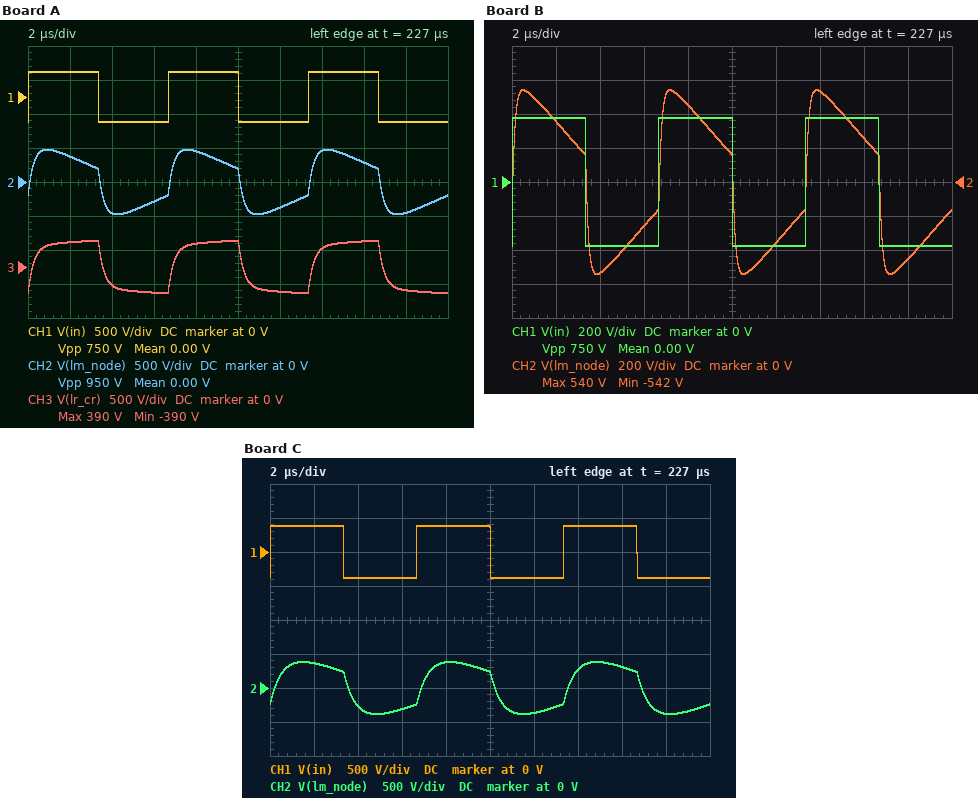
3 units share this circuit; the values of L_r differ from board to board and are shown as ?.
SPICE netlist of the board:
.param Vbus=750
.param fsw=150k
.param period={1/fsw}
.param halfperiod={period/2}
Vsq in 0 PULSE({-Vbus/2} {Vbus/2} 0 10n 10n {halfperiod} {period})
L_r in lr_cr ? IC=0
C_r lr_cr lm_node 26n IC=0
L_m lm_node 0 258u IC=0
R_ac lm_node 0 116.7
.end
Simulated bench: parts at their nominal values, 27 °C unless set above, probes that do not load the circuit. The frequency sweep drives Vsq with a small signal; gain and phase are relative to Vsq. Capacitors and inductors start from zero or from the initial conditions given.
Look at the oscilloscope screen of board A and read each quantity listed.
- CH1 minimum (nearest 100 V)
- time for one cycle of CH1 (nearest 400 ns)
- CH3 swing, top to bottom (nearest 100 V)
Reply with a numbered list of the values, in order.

1. -400 V
2. 6.8 µs
3. 800 V
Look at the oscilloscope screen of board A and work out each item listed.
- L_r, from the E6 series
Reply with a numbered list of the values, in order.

1. 33 µH
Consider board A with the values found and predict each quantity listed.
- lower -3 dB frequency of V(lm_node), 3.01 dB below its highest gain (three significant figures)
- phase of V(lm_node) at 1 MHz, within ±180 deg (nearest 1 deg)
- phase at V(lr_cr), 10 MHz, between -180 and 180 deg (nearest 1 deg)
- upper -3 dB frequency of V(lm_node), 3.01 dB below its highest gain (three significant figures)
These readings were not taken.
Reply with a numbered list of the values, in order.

1. 50.4 kHz
2. -57 deg
3. -87 deg
4. 185 kHz
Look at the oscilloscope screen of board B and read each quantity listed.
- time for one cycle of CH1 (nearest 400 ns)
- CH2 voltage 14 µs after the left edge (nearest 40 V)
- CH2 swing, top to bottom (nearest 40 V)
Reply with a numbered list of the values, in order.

1. 6.8 µs
2. 520 V
3. 1.08 kV
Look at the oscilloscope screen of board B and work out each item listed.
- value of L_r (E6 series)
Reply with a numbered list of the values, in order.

1. 15 µH
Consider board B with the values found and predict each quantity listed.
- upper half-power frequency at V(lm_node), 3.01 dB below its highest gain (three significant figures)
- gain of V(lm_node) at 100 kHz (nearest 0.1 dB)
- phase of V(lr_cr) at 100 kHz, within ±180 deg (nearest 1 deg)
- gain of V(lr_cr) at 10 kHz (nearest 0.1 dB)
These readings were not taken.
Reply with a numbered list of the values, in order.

1. 410 kHz
2. 1.8 dB
3. -7 deg
4. 0 dB
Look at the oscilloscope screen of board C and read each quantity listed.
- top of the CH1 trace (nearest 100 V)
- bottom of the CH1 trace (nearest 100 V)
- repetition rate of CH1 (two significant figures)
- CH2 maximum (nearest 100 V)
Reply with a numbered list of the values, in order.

1. 400 V
2. -400 V
3. 150 kHz
4. 400 V
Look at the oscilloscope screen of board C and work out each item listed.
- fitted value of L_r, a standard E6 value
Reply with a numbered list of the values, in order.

1. 68 µH
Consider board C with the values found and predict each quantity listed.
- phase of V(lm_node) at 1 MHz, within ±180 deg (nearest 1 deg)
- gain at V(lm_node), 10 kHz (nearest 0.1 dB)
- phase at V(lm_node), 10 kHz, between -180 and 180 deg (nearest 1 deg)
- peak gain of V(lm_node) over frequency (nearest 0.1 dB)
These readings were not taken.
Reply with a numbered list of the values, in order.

1. -71 deg
2. -31.3 dB
3. 172 deg
4. 3.4 dB
